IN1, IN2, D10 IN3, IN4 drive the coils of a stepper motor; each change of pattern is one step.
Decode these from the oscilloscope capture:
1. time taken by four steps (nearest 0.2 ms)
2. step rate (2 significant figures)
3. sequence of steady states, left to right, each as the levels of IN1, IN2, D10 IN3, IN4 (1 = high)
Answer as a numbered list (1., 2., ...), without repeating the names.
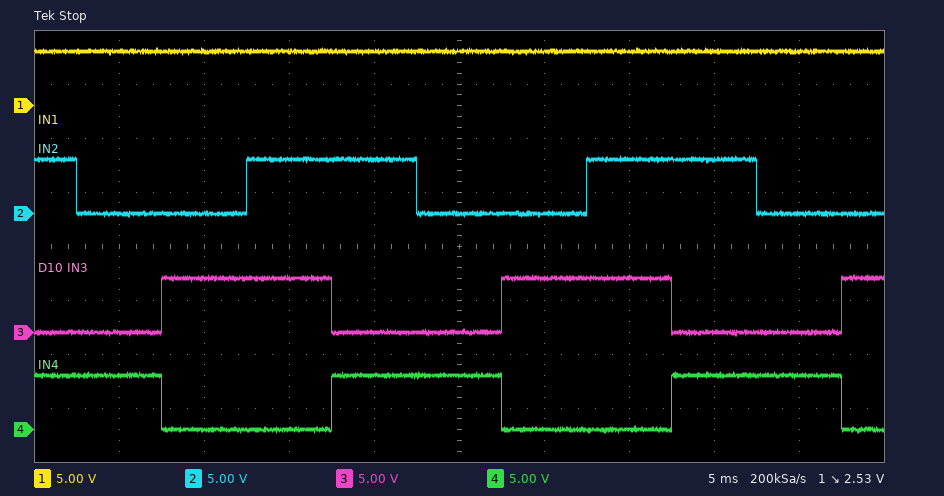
1. 20.0 ms
2. 200 steps/s
3. 1101 1001 1010 1110 1101 1001 1010 1110 1101 1001 1010
